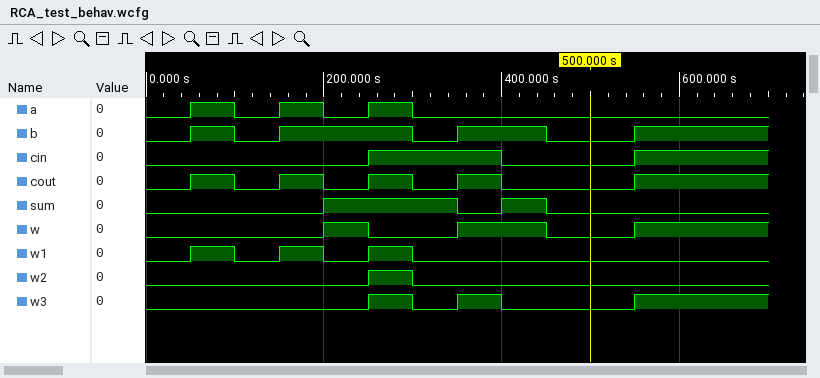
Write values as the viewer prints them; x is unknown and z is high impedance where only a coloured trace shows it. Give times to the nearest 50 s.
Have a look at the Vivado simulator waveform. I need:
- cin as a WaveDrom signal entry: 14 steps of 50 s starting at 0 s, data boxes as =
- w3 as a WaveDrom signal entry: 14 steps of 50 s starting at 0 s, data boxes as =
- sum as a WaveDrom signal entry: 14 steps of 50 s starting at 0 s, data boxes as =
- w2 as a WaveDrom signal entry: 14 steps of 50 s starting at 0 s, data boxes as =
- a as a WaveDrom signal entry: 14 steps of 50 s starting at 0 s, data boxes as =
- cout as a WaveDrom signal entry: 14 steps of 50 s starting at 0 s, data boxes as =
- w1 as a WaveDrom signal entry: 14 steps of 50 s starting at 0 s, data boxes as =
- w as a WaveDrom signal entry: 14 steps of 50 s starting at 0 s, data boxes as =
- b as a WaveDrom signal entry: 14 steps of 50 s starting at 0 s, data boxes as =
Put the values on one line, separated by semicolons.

{name: 'cin', wave: '0....1..0..1..'}; {name: 'w3', wave: '0....1010..1..'}; {name: 'sum', wave: '0...1..010....'}; {name: 'w2', wave: '0....10.......'}; {name: 'a', wave: '0101010.......'}; {name: 'cout', wave: '010101010..1..'}; {name: 'w1', wave: '0101010.......'}; {name: 'w', wave: '0...10.1.0.1..'}; {name: 'b', wave: '0101..01.0.1..'}
